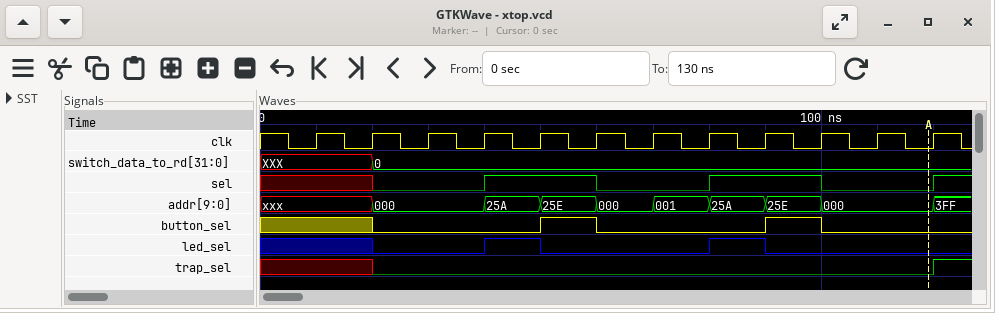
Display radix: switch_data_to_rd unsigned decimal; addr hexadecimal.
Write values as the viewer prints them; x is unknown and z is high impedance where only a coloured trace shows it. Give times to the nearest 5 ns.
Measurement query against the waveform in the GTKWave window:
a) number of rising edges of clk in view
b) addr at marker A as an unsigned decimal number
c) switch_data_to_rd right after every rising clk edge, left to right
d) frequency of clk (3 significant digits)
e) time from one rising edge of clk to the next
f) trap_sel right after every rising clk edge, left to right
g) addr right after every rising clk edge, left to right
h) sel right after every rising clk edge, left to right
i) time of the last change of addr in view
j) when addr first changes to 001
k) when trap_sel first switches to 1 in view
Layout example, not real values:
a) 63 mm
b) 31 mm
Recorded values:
a) 12
b) 0
c) XXX, 0, 0, 0, 0, 0, 0, 0, 0, 0, 0, 0
d) 100 MHz
e) 10 ns
f) x 0 0 0 0 0 0 0 0 0 0 1
g) xxx, 000, 000, 25A, 25E, 000, 001, 25A, 25E, 000, 000, 3FF
h) x 0 0 1 1 0 0 1 1 0 0 1
i) 120 ns
j) 70 ns
k) 120 ns
